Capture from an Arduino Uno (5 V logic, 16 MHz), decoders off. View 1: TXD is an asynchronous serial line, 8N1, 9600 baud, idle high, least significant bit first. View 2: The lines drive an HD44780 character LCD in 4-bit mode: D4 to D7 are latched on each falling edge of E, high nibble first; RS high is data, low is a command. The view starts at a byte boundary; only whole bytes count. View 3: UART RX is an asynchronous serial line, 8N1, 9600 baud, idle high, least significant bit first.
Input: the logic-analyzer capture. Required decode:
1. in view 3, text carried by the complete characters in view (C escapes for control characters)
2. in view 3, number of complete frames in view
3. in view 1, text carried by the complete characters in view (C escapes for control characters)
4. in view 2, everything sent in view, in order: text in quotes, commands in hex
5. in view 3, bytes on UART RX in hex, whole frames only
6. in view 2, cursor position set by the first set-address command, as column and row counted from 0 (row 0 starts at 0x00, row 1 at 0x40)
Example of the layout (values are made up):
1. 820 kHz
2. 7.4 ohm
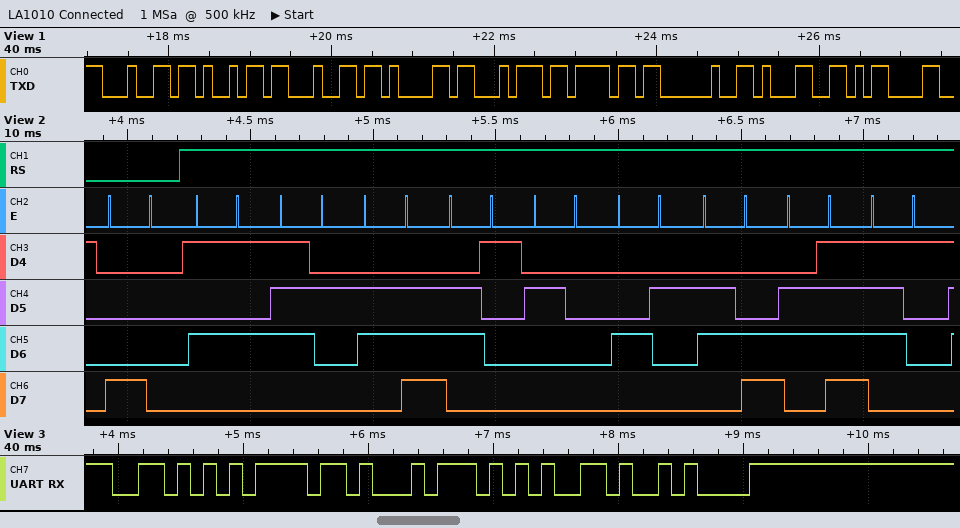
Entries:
1. "Vote\n"
2. 5
3. "didato 1\r"
4. 0x80 "Urna Bloq"
5. 56 6F 74 65 0A
6. column 0, row 0
